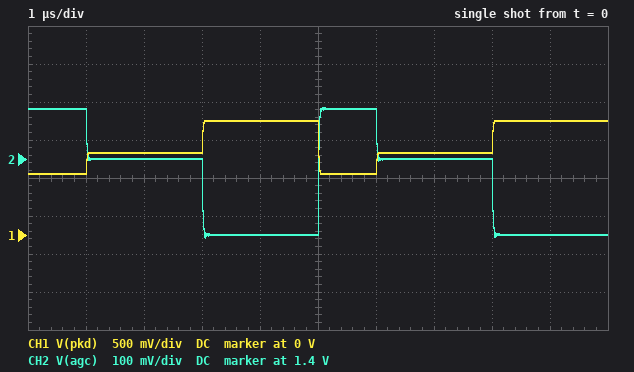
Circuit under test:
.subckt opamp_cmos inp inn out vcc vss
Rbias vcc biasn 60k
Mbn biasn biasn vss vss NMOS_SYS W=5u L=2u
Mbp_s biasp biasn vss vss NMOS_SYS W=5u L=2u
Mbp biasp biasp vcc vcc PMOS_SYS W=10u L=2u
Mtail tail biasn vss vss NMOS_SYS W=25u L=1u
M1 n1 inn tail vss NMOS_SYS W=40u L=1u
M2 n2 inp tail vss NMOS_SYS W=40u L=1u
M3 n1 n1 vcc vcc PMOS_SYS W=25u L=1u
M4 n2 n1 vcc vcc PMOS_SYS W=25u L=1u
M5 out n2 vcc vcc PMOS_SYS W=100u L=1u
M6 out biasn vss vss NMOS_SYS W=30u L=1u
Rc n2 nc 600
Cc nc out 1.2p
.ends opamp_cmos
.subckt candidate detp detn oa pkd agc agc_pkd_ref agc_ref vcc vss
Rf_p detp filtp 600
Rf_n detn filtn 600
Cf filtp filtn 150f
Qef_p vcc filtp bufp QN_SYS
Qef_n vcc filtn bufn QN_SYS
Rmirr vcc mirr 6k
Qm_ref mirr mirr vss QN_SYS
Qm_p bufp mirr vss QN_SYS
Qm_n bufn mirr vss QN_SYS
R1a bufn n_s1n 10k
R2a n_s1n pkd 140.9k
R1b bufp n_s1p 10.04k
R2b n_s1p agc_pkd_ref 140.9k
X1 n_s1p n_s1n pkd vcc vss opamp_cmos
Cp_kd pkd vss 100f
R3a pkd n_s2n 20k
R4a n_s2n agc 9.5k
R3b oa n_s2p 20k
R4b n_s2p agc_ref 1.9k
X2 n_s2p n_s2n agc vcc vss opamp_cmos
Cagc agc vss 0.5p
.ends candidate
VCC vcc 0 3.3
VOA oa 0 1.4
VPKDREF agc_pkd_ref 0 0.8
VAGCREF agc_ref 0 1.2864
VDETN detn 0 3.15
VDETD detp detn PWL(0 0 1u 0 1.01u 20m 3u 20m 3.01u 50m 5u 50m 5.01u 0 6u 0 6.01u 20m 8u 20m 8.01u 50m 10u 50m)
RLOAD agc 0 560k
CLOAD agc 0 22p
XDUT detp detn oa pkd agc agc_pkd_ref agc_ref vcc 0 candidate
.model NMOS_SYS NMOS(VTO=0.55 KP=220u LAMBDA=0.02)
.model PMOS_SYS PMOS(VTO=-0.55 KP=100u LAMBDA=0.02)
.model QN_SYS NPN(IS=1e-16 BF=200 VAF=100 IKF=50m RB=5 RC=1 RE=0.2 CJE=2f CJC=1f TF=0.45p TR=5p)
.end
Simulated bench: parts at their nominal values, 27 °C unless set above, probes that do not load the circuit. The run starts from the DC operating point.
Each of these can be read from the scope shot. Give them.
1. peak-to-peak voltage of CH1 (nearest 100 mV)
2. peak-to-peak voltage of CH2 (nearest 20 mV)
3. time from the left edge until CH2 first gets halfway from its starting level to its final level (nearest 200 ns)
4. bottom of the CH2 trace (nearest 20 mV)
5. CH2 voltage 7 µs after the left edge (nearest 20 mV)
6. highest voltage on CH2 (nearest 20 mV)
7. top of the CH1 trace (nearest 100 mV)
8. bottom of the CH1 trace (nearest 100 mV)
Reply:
700 mV
340 mV
3.0 µs
1.20 V
1.40 V
1.54 V
1.5 V
800 mV
